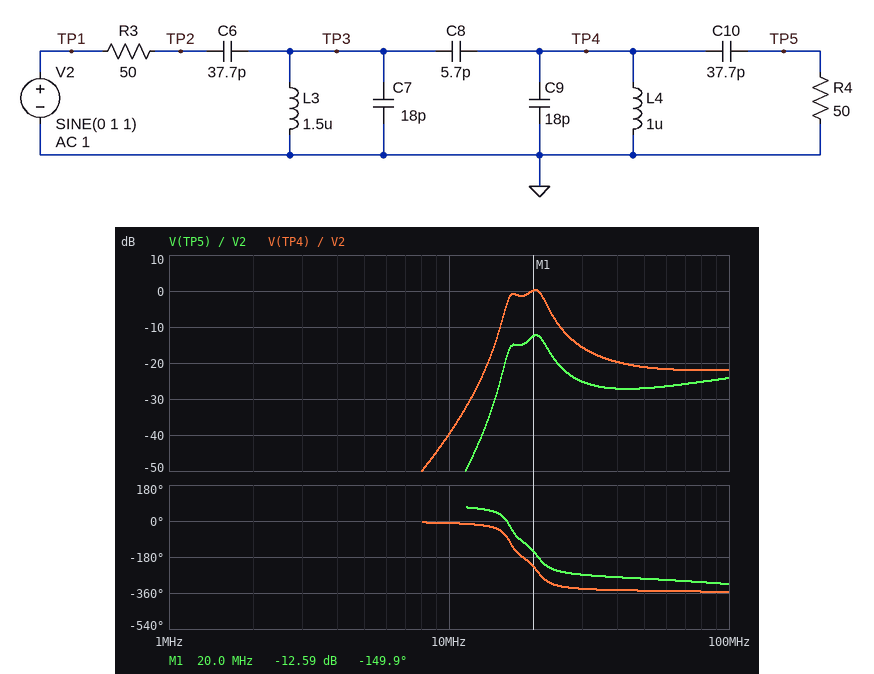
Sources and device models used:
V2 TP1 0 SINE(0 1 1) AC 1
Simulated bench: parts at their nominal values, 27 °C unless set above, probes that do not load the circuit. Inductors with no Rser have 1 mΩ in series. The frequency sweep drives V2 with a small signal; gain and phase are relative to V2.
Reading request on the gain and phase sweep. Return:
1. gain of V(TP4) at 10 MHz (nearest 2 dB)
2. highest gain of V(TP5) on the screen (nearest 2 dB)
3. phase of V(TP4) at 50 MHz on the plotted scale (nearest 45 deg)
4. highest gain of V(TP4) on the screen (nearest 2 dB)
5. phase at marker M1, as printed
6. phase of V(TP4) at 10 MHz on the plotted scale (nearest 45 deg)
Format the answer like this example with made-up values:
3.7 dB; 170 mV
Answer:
-40 dB; -12 dB; -360 deg; 0 dB; -149.9 deg; 0 deg
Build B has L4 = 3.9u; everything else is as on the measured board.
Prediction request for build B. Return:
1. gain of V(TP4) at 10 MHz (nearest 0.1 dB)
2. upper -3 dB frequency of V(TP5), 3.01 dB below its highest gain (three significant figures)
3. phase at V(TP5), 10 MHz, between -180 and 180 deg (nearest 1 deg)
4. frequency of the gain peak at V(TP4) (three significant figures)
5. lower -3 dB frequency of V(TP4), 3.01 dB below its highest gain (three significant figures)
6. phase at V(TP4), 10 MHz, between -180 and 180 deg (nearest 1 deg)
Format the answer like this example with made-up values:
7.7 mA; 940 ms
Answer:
-9.4 dB; 18.0 MHz; 25 deg; 16.8 MHz; 15.7 MHz; -59 deg
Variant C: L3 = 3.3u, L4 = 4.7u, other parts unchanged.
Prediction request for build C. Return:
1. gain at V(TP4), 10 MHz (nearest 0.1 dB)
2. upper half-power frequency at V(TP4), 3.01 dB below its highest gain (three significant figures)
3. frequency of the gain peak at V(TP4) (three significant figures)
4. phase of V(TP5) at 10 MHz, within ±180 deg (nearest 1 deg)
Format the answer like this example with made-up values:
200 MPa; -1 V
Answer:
2.1 dB; 11.8 MHz; 11.3 MHz; -90 deg
